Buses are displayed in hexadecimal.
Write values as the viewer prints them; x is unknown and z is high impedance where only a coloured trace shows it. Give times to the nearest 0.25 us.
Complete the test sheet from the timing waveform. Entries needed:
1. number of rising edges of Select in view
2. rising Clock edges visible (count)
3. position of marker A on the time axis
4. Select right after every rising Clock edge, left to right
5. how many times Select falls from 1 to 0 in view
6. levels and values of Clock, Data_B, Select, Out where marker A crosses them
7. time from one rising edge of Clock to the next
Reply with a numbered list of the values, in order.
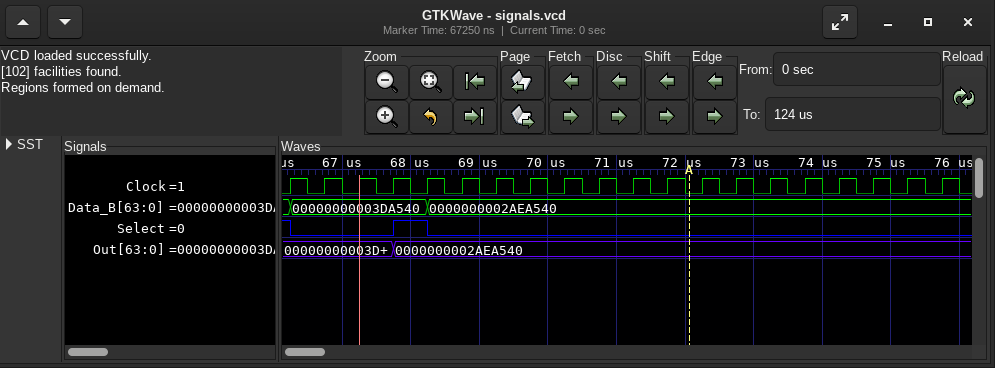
1. 1
2. 20
3. 72 us
4. 0 0 0 1 0 0 0 0 0 0 0 0 0 0 0 0 0 0 0 0
5. 2
6. Clock=0, Data_B=0000000002AEA540, Select=0, Out=0000000002AEA540
7. 0.5 us
